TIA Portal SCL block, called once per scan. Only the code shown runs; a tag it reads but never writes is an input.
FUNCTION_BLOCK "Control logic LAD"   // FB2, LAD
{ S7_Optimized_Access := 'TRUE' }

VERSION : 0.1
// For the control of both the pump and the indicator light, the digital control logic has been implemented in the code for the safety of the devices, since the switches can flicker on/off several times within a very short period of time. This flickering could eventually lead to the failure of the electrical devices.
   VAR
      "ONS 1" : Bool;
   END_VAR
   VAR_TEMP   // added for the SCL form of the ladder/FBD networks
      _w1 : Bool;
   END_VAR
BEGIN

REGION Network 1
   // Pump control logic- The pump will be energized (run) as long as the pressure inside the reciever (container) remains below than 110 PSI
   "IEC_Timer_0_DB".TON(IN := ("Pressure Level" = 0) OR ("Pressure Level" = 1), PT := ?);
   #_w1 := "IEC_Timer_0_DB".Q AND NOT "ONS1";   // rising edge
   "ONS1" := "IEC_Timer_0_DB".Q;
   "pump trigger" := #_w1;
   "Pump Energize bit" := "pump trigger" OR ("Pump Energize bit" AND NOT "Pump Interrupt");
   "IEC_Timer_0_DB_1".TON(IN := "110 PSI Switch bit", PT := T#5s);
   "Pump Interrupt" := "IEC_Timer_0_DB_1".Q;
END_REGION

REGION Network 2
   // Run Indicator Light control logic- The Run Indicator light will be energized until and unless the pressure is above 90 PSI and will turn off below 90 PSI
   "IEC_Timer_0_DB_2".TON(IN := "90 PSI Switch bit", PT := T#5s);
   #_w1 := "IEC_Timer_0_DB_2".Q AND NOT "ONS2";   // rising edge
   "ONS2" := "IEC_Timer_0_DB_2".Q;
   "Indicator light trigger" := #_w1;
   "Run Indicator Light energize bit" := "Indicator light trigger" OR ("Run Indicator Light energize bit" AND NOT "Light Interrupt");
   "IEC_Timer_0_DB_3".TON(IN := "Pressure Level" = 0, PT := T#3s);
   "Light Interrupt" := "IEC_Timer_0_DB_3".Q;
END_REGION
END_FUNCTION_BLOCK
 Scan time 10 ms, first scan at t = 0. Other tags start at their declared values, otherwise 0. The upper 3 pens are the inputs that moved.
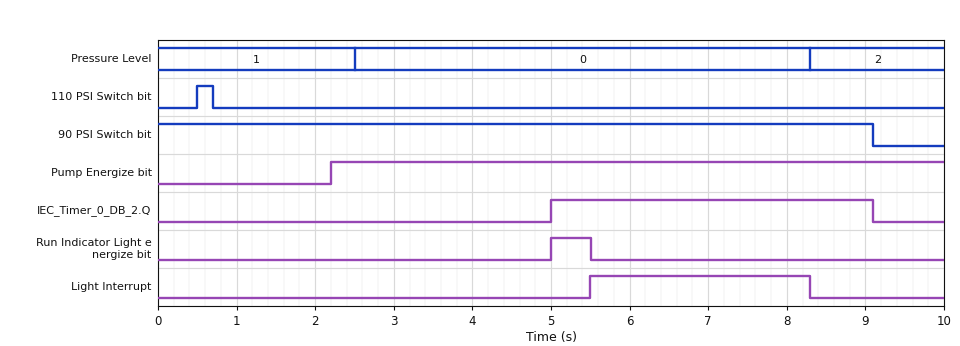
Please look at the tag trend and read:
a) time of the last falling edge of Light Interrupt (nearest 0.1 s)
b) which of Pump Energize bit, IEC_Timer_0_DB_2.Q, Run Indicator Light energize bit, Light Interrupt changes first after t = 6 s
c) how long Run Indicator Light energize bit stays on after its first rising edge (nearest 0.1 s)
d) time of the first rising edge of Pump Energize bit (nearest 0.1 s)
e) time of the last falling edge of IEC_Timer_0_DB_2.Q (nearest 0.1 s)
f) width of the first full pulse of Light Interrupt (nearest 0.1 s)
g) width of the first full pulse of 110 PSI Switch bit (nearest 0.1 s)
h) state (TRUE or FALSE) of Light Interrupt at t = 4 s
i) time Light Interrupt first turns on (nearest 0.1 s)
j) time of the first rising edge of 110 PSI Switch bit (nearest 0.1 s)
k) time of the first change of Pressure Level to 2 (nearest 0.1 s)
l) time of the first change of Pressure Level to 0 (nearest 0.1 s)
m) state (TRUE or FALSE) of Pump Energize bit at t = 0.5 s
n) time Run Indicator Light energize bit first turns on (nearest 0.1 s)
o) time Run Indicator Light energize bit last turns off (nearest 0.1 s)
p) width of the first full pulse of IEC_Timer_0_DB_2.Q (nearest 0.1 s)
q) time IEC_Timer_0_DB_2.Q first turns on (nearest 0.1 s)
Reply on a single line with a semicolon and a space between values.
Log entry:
8.3 s; Light Interrupt; 0.5 s; 2.2 s; 9.1 s; 2.8 s; 0.2 s; FALSE; 5.5 s; 0.5 s; 8.3 s; 2.5 s; FALSE; 5.0 s; 5.5 s; 4.1 s; 5.0 s
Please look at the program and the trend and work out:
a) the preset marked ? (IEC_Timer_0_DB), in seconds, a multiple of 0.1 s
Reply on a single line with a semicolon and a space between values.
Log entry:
2.2 s
